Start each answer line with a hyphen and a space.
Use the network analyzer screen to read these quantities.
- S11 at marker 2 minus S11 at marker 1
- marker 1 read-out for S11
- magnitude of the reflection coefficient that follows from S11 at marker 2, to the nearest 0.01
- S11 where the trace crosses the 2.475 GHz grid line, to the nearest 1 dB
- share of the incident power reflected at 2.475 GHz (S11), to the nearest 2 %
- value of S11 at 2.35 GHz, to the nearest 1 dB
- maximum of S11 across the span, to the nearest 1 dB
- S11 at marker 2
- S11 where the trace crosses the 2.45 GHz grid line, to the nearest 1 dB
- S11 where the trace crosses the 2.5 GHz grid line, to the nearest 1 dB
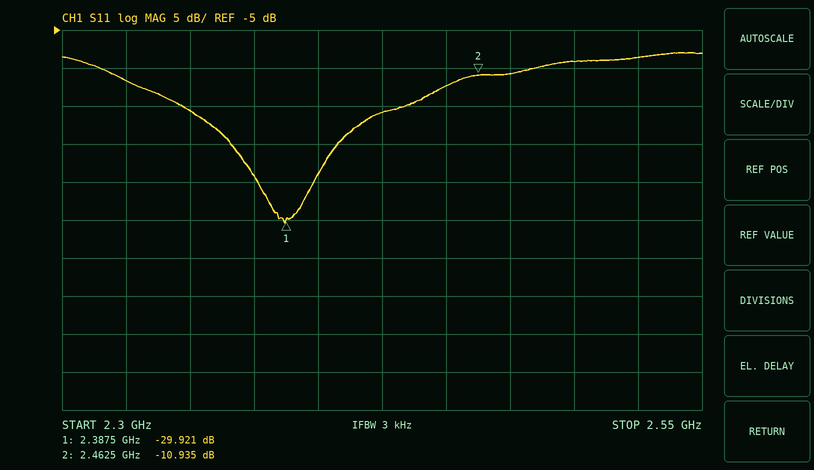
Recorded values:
- 18.986 dB
- -29.921 dB
- 0.28
- -11 dB
- 8 %
- -16 dB
- -8 dB
- -10.935 dB
- -12 dB
- -9 dB
